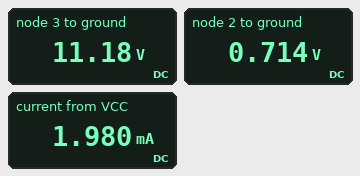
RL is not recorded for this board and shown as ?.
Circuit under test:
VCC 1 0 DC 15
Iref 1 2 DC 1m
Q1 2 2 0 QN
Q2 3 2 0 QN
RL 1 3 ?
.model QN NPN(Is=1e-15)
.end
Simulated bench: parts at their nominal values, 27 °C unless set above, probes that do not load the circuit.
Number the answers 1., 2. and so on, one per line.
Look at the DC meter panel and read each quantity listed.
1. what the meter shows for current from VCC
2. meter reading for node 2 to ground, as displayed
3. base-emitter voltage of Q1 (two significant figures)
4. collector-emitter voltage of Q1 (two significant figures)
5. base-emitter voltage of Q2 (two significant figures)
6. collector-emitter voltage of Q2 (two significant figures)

1. 1.980 mA
2. 0.714 V
3. 710 mV
4. 710 mV
5. 710 mV
6. 11 V
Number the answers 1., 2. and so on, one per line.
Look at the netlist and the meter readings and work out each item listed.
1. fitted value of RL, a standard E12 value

1. 3.9 kΩ
